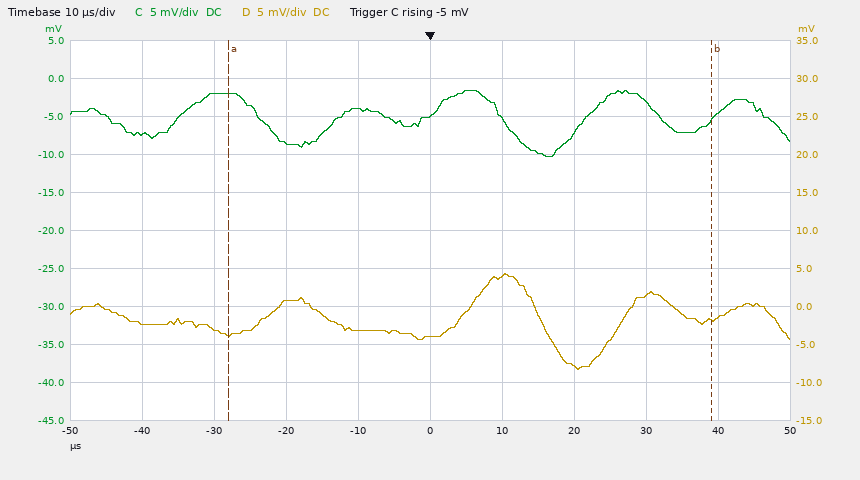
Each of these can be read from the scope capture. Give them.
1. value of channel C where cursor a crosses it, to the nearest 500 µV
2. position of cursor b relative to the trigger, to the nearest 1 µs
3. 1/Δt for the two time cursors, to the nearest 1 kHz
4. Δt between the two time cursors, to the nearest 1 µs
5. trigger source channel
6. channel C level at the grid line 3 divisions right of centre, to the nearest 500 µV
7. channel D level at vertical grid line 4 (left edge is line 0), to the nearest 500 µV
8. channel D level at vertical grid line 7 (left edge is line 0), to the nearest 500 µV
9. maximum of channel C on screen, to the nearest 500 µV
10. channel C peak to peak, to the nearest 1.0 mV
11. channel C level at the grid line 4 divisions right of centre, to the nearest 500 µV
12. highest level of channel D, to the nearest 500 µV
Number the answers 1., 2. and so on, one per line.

1. -2.0 mV
2. +39 µs
3. 15 kHz
4. 67 µs
5. channel C
6. -3.0 mV
7. -3.0 mV
8. -8.0 mV
9. -1.5 mV
10. 9.0 mV
11. -4.5 mV
12. 4.5 mV
